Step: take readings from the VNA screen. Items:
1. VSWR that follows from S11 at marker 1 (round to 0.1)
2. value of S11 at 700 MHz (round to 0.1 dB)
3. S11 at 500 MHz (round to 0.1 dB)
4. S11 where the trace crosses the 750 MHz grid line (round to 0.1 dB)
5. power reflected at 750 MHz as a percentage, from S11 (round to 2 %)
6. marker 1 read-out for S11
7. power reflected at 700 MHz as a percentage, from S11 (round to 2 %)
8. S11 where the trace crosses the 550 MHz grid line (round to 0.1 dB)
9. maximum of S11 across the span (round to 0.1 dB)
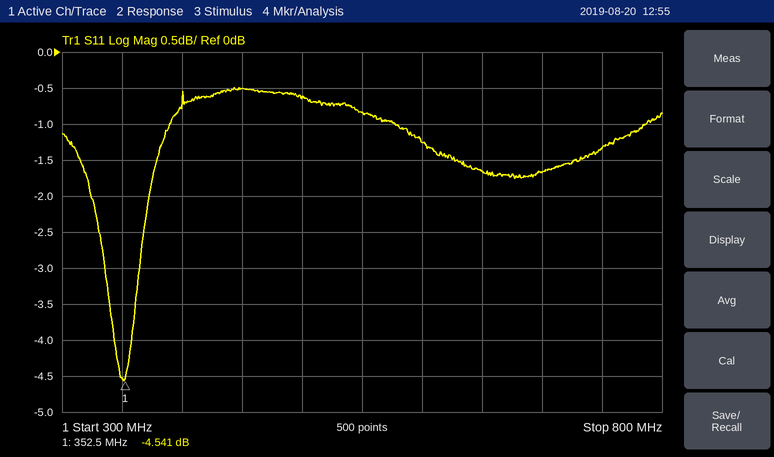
3.9
-1.7 dB
-0.6 dB
-1.3 dB
74 %
-4.541 dB
68 %
-0.8 dB
-0.5 dB
